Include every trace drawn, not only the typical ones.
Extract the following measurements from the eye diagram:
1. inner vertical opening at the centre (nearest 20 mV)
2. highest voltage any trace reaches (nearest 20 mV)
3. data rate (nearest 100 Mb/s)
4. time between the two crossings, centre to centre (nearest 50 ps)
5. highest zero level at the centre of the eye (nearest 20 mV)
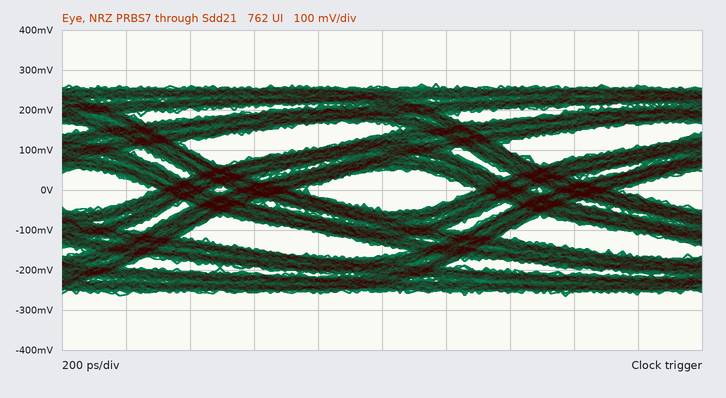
100 mV
260 mV
1.0 Gb/s
1.00 ns
-60 mV
